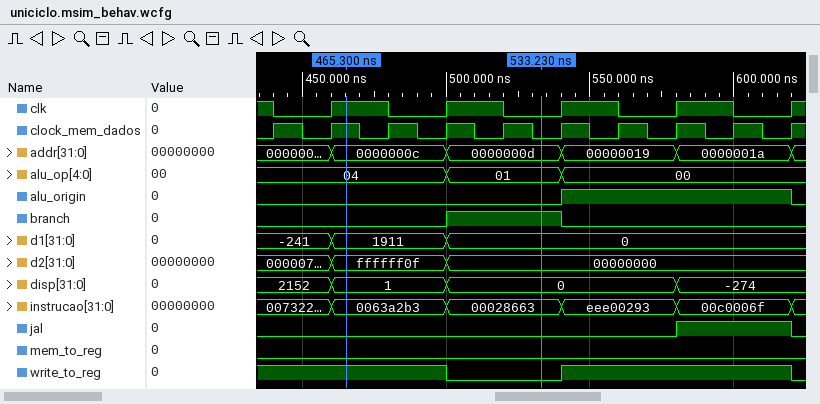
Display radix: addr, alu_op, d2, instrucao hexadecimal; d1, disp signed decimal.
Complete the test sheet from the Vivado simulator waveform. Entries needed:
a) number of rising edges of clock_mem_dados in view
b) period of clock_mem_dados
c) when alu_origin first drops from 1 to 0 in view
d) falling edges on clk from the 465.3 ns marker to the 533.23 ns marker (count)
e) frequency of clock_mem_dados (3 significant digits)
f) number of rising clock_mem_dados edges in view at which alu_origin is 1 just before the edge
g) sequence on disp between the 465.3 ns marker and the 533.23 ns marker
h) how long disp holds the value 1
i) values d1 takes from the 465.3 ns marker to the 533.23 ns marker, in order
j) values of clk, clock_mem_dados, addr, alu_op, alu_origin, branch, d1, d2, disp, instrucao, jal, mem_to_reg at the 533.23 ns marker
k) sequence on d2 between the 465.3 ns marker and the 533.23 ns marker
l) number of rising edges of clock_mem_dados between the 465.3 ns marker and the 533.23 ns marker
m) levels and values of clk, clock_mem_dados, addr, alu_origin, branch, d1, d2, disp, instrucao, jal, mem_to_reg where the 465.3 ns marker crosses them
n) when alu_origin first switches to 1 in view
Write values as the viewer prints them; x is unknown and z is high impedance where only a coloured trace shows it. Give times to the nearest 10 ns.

10
20 ns
620 ns
2
50.0 MHz
4
1, 0
40 ns
1911, 0
clk=0, clock_mem_dados=0, addr=0000000d, alu_op=01, alu_origin=0, branch=1, d1=0, d2=00000000, disp=0, instrucao=00028663, jal=0, mem_to_reg=0
ffffff0f, 00000000
3
clk=1, clock_mem_dados=1, addr=0000000c, alu_origin=0, branch=0, d1=1911, d2=ffffff0f, disp=1, instrucao=0063a2b3, jal=0, mem_to_reg=0
540 ns
